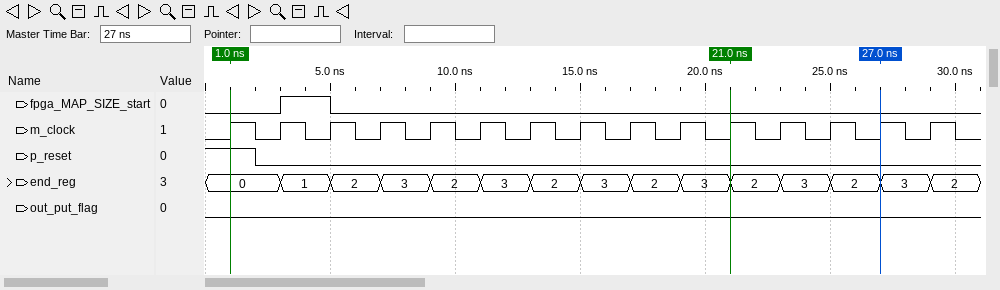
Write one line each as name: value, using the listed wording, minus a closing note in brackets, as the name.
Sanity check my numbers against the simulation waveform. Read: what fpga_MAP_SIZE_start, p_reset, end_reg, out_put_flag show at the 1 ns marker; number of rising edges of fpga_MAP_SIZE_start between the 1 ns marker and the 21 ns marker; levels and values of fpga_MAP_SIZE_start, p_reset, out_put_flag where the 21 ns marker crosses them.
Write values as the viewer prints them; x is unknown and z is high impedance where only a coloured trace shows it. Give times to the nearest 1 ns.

what fpga_MAP_SIZE_start, p_reset, end_reg, out_put_flag show at the 1 ns marker: fpga_MAP_SIZE_start=0, p_reset=1, end_reg=0, out_put_flag=0
number of rising edges of fpga_MAP_SIZE_start between the 1 ns marker and the 21 ns marker: 1
levels and values of fpga_MAP_SIZE_start, p_reset, out_put_flag where the 21 ns marker crosses them: fpga_MAP_SIZE_start=0, p_reset=0, out_put_flag=0
